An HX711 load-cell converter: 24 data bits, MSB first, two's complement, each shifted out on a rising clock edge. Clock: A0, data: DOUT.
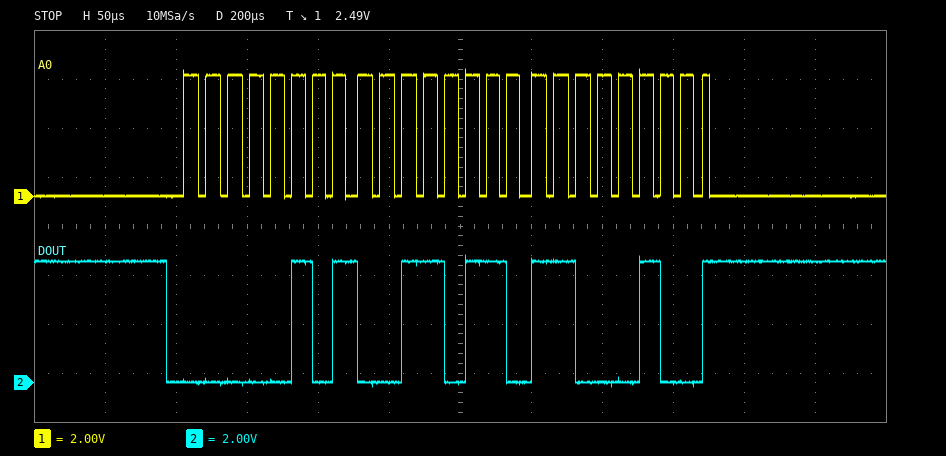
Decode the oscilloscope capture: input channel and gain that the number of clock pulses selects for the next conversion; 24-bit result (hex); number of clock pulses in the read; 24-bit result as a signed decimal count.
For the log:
channel A, gain 128
0x0536C4
25
341700
